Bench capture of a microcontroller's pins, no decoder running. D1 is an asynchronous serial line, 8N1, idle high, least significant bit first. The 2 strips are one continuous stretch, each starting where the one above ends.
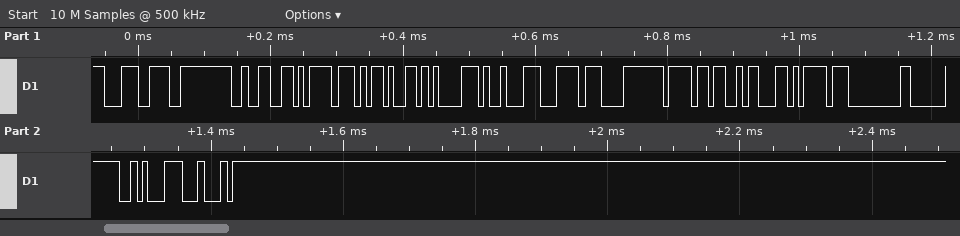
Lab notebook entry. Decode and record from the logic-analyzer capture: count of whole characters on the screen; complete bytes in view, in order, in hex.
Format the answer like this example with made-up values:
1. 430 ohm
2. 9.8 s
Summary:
1. 16
2. 0x9C 0xFE 0x32 0xBD 0x2D 0x85 0x89 0xBC 0xF8 0x6F 0x1A 0xBD 0x00 0xE0 0x8A 0x44
